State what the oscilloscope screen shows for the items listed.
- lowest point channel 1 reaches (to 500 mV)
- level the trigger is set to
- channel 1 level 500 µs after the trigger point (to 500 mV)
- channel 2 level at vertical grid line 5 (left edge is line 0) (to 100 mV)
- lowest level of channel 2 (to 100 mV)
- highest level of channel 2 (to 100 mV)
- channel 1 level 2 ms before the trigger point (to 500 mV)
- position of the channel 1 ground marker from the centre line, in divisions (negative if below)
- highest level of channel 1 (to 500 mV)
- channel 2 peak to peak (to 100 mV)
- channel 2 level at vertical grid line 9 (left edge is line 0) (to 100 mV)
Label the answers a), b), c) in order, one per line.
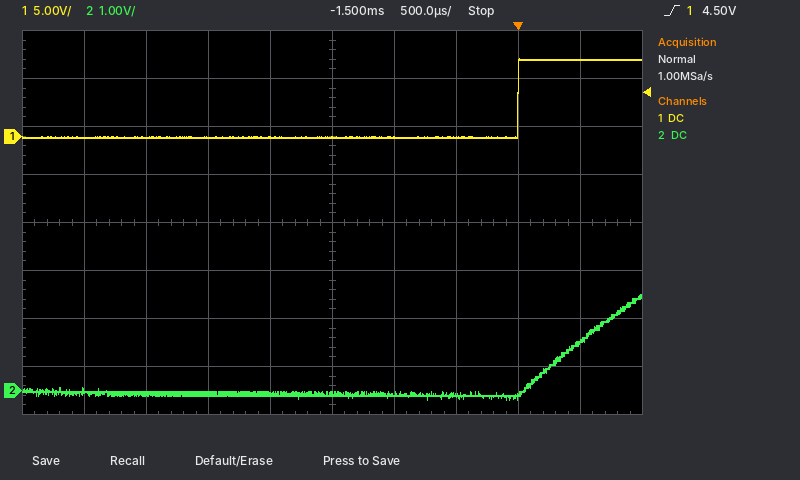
a) 0.0 V
b) 4.50 V
c) 8.0 V
d) -100 mV
e) -200 mV
f) 2.0 V
g) 0.0 V
h) +1.8 div
i) 8.0 V
j) 2.2 V
k) 1.0 V
